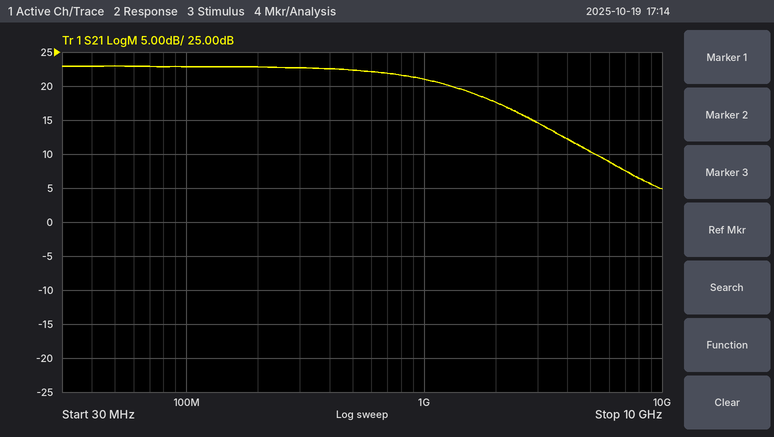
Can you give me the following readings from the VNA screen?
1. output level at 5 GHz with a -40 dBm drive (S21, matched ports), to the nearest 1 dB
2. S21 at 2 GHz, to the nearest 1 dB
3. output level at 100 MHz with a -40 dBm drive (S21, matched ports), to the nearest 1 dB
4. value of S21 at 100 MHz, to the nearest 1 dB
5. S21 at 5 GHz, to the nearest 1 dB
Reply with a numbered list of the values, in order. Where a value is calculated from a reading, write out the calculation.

1. -40 dBm + (10 dB) = -30 dBm
2. 18 dB
3. -40 dBm + (23 dB) = -17 dBm
4. 23 dB
5. 10 dB
